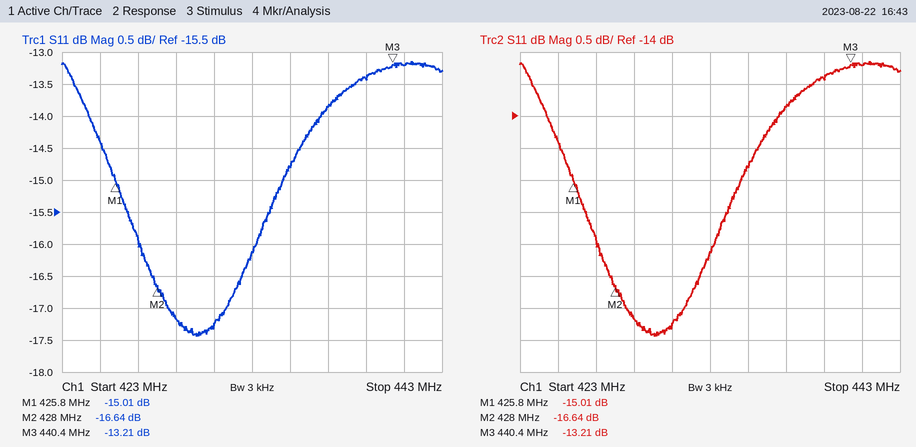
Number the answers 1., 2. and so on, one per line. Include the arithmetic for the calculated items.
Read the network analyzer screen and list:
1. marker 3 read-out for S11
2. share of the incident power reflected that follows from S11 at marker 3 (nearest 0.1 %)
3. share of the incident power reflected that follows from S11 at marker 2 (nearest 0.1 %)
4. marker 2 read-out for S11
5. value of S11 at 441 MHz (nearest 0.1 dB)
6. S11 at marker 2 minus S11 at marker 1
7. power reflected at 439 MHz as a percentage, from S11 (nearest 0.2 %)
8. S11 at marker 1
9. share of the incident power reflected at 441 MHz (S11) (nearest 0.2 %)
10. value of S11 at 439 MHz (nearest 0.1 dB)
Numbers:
1. -13.21 dB
2. 10^(-13.21/10) ≈ 4.8 %
3. 10^(-16.64/10) ≈ 2.2 %
4. -16.64 dB
5. -13.2 dB
6. -16.64 − (-15.01) = -1.63 dB
7. 10^(-13.4/10) ≈ 4.6 %
8. -15.01 dB
9. 10^(-13.2/10) ≈ 4.8 %
10. -13.4 dB
